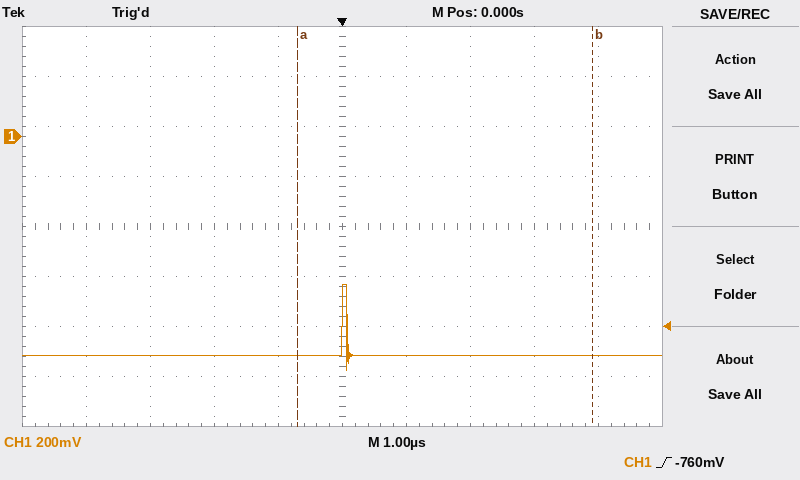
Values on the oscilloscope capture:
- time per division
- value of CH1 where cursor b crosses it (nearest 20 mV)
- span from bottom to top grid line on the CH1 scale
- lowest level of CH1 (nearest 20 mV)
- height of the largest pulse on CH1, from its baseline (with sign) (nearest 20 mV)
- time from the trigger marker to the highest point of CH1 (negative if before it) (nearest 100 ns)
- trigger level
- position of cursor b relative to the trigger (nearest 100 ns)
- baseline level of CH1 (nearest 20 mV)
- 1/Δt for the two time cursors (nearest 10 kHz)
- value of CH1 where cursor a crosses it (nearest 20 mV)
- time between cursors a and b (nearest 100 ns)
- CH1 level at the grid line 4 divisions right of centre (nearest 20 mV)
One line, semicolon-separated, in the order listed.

1 µs; -880 mV; 1.6 V; -940 mV; +280 mV; 0.0 µs; -760 mV; +3.9 µs; -880 mV; 220 kHz; -880 mV; 4.6 µs; -880 mV
